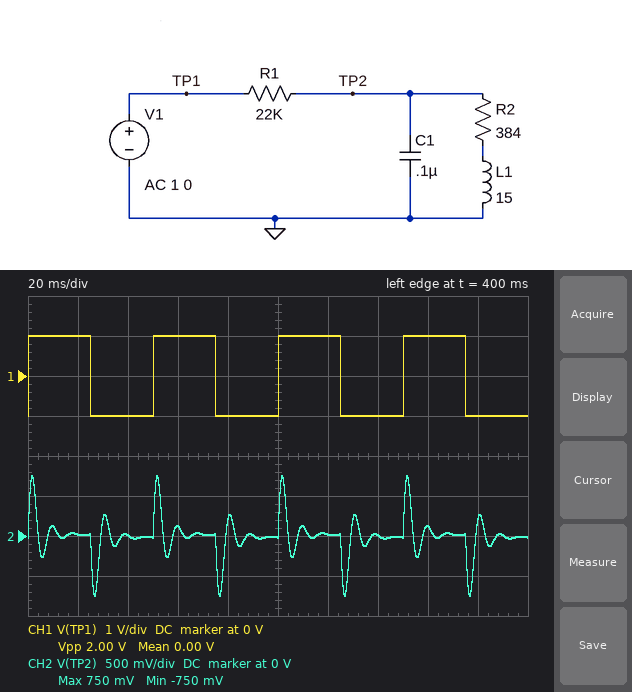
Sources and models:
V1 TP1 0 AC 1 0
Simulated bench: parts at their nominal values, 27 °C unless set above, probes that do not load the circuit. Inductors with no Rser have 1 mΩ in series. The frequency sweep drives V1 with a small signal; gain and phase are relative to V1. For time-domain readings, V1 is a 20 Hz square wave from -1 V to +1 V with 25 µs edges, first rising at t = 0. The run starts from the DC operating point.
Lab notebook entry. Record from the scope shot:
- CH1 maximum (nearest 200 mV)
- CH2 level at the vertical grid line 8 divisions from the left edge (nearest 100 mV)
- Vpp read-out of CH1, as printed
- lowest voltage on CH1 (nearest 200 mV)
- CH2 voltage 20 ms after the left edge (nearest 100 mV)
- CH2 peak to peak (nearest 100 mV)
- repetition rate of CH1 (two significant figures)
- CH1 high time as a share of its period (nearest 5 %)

1.0 V
100 mV
2.00 V
-1.0 V
0 V
1.5 V
20 Hz
50 %
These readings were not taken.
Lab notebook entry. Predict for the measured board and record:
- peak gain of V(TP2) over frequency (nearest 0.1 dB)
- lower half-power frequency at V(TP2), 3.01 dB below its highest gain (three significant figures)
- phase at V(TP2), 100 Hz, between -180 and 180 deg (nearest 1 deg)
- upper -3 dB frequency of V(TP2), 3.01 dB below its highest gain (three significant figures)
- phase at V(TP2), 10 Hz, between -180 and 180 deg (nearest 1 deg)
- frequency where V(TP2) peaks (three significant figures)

-0.5 dB
98.3 Hz
41 deg
175 Hz
65 deg
131 Hz
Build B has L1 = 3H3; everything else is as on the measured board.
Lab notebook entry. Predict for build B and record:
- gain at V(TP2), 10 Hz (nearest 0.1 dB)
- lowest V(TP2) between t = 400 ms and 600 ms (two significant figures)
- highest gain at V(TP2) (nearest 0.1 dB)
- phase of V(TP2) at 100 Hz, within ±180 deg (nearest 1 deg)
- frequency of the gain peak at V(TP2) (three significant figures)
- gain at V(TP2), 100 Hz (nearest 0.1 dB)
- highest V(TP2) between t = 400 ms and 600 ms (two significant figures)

-34.2 dB
-420 mV
-2.0 dB
72 deg
279 Hz
-19.4 dB
420 mV
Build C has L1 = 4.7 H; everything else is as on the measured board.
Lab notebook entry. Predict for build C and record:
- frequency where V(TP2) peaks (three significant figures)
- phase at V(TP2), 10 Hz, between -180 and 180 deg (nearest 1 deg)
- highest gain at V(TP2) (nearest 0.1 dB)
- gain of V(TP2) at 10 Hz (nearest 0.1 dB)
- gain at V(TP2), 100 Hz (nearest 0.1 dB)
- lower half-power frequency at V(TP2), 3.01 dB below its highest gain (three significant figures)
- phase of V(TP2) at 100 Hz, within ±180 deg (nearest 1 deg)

234 Hz
37 deg
-1.4 dB
-33.3 dB
-15.9 dB
195 Hz
72 deg
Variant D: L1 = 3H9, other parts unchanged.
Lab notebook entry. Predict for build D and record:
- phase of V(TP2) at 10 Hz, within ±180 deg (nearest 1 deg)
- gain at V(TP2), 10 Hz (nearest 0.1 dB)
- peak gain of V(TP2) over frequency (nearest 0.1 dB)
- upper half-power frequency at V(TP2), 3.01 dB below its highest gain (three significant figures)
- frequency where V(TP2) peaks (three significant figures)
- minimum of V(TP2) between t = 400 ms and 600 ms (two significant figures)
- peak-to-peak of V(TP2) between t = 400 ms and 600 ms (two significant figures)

32 deg
-33.8 dB
-1.7 dB
305 Hz
257 Hz
-450 mV
900 mV
